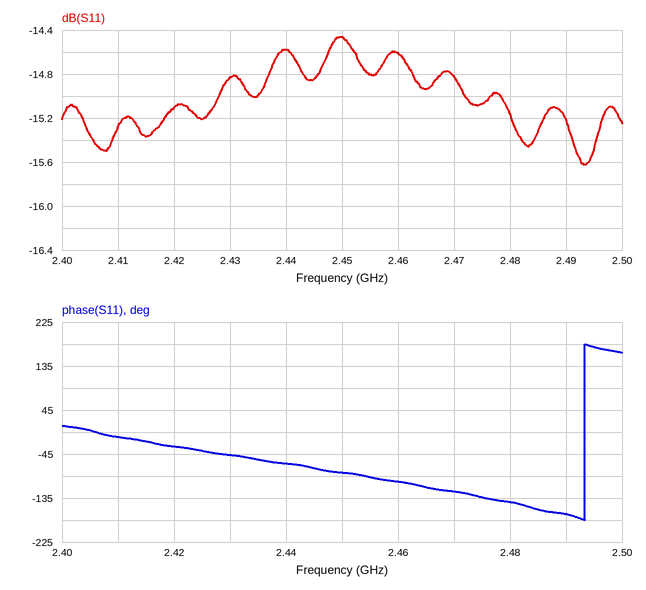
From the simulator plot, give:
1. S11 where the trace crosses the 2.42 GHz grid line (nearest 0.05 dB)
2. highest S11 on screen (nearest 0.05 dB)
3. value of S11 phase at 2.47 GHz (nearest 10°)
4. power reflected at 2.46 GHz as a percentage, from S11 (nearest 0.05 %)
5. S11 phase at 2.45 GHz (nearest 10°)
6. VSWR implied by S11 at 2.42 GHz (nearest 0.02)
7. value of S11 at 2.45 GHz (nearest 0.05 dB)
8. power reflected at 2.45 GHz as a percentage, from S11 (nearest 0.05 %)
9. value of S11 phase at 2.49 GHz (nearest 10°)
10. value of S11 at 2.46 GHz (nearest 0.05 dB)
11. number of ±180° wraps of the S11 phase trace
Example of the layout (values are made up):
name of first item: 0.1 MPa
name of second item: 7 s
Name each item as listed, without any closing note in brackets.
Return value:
S11 where the trace crosses the 2.42 GHz grid line: -15.10 dB
highest S11 on screen: -14.45 dB
value of S11 phase at 2.47 GHz: -120°
power reflected at 2.46 GHz as a percentage, from S11: 3.45 %
S11 phase at 2.45 GHz: -80°
VSWR implied by S11 at 2.42 GHz: 1.42
value of S11 at 2.45 GHz: -14.45 dB
power reflected at 2.45 GHz as a percentage, from S11: 3.60 %
value of S11 phase at 2.49 GHz: -170°
value of S11 at 2.46 GHz: -14.60 dB
number of ±180° wraps of the S11 phase trace: 1
